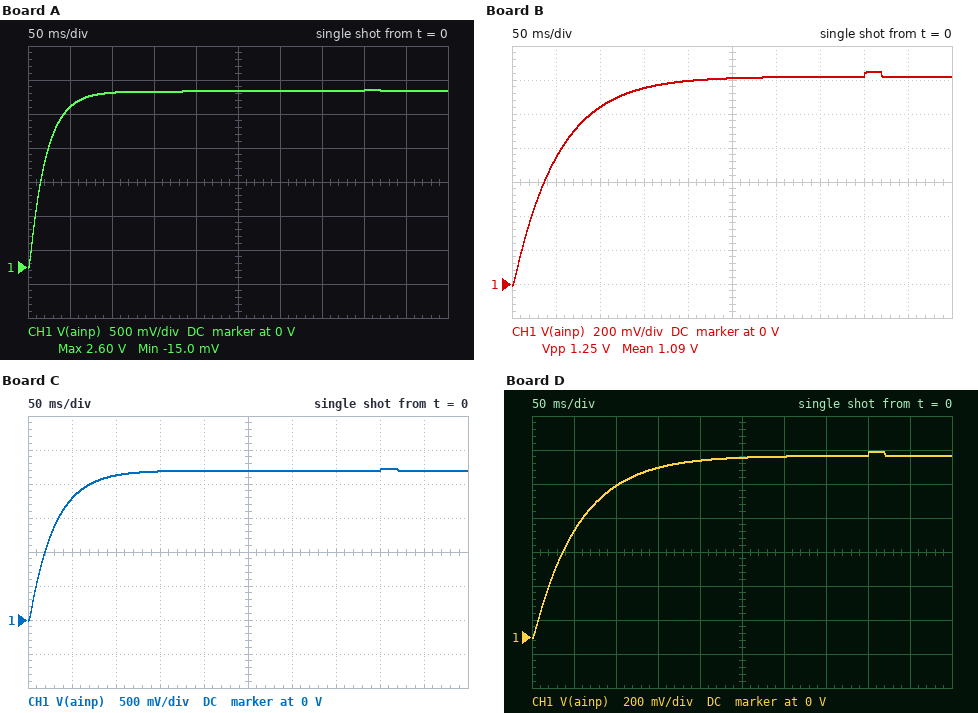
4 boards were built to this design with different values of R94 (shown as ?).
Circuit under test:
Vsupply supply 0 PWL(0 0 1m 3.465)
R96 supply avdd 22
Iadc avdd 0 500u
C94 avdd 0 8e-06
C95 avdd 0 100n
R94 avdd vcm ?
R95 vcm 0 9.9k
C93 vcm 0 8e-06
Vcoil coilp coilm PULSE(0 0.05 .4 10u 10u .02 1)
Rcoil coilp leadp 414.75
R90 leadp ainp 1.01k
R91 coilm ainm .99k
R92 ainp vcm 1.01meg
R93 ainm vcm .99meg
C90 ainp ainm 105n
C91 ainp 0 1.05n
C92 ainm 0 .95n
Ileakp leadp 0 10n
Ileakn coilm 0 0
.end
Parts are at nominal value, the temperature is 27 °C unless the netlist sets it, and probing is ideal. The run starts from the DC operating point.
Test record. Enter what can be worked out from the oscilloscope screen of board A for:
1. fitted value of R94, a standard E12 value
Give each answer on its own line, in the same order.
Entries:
3.3 kΩ
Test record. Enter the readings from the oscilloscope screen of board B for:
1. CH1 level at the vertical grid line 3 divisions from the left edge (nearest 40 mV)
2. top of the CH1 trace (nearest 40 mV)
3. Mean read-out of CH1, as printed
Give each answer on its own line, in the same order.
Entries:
1.16 V
1.24 V
1.09 V
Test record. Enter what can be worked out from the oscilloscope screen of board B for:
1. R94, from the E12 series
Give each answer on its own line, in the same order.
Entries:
18 kΩ
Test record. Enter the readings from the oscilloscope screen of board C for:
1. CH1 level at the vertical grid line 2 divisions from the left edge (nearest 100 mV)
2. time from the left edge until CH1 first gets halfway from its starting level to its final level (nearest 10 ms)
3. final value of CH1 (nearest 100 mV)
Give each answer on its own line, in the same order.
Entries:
2.1 V
20 ms
2.2 V
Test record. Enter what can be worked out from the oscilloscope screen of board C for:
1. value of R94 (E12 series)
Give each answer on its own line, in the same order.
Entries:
5.6 kΩ
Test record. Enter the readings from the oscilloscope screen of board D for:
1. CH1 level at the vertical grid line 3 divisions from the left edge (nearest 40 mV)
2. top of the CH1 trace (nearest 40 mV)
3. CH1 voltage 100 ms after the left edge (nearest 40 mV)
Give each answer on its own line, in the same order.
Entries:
1.00 V
1.08 V
880 mV
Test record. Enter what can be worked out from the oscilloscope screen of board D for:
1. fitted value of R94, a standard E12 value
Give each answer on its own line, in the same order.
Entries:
22 kΩ
